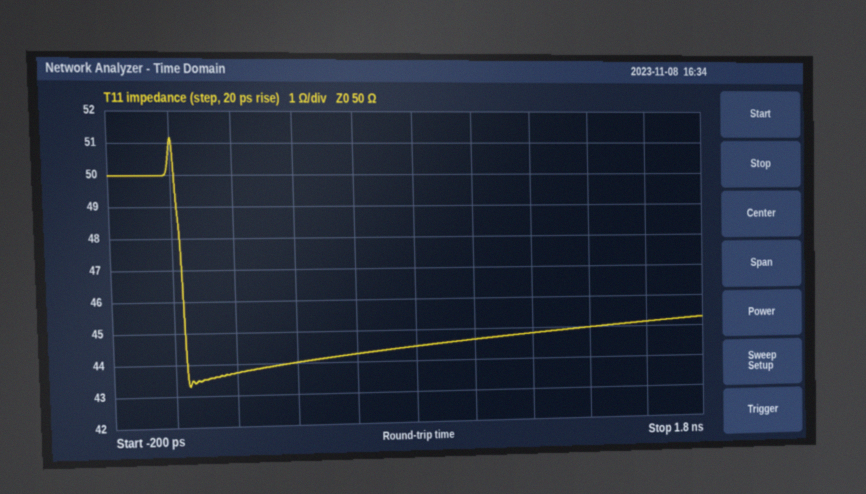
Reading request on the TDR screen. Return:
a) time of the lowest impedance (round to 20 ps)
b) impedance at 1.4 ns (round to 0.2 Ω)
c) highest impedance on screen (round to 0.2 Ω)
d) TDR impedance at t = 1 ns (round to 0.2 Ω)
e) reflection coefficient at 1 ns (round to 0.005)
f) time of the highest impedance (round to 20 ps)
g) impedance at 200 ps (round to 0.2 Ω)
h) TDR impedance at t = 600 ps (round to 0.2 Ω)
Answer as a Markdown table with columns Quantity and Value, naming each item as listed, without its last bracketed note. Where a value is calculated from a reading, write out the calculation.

| Quantity | Value |
|---|---|
| time of the lowest impedance | 40 ps |
| impedance at 1.4 ns | 45.0 Ω |
| highest impedance on screen | 51.2 Ω |
| TDR impedance at t = 1 ns | 44.6 Ω |
| reflection coefficient at 1 ns | (44.6 − 50)/(44.6 + 50) ≈ -0.0571, so -0.055 to the nearest 0.005 |
| time of the highest impedance | 0 ps |
| impedance at 200 ps | 43.8 Ω |
| TDR impedance at t = 600 ps | 44.2 Ω |
